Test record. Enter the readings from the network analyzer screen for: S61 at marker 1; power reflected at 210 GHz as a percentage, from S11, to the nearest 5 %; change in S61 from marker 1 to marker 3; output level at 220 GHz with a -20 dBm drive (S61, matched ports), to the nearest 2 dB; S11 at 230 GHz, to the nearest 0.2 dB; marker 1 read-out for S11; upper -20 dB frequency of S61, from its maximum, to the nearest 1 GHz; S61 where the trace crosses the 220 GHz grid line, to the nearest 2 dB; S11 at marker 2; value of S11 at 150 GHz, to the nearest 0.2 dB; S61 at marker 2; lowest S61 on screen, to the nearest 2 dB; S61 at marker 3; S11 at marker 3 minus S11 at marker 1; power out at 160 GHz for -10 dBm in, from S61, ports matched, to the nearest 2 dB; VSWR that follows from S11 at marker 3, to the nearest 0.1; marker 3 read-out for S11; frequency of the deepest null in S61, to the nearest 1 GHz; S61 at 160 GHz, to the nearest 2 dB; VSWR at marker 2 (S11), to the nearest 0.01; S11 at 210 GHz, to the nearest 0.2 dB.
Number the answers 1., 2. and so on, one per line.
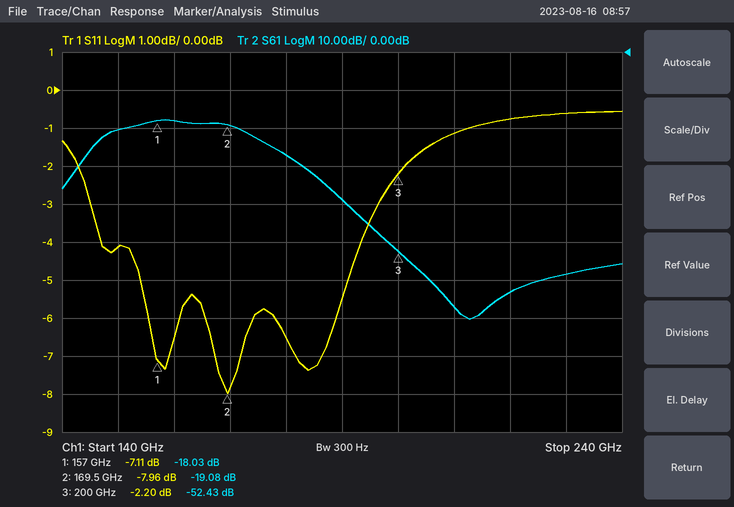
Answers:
1. -18.03 dB
2. 75 %
3. -34.40 dB
4. -84 dBm
5. -0.6 dB
6. -7.11 dB
7. 189 GHz
8. -64 dB
9. -7.96 dB
10. -4.2 dB
11. -19.08 dB
12. -70 dB
13. -52.43 dB
14. 4.91 dB
15. -28 dBm
16. 7.9
17. -2.20 dB
18. 213 GHz
19. -18 dB
20. 2.33
21. -1.2 dB
